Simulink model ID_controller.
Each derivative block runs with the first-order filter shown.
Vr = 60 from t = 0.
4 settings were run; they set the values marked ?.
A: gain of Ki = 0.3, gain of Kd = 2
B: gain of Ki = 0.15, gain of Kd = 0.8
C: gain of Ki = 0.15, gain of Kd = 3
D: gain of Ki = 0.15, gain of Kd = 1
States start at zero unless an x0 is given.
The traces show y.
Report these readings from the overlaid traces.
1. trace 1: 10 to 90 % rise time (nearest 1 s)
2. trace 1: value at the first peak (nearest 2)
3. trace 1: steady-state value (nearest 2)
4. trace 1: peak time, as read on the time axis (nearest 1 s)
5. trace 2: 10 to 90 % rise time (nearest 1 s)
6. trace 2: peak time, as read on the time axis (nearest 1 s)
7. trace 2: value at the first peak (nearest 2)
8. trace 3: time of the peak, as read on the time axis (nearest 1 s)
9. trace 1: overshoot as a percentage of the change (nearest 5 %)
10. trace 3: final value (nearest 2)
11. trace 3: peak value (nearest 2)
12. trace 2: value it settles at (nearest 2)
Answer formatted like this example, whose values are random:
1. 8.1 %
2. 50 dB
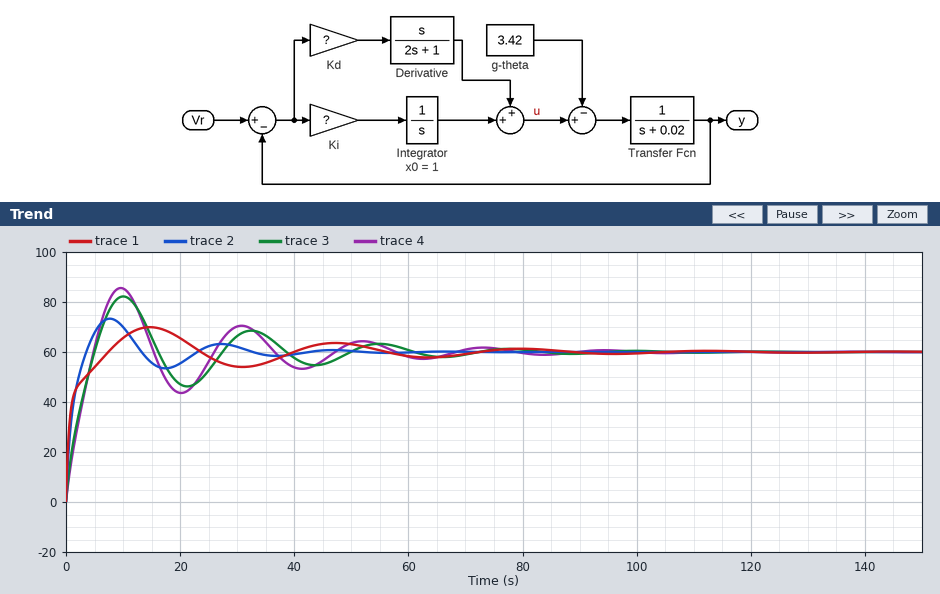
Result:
1. 5 s
2. 70
3. 60
4. 15 s
5. 3 s
6. 8 s
7. 74
8. 10 s
9. 15 %
10. 60
11. 82
12. 60
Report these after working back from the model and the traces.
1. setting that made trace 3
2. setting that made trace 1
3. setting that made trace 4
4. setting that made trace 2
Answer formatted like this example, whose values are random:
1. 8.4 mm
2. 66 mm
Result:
1. D
2. C
3. B
4. A
